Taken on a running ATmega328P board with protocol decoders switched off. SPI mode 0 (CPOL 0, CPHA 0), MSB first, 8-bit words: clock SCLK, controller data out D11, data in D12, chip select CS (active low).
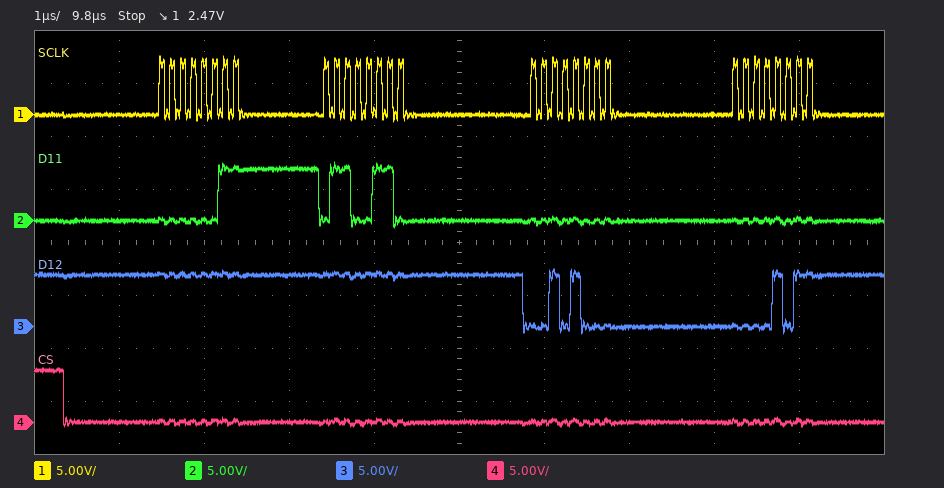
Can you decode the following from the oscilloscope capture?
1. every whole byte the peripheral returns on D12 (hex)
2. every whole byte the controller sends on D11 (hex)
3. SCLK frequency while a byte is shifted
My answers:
FF FF 28 0B
03 66 00 00
8 MHz
